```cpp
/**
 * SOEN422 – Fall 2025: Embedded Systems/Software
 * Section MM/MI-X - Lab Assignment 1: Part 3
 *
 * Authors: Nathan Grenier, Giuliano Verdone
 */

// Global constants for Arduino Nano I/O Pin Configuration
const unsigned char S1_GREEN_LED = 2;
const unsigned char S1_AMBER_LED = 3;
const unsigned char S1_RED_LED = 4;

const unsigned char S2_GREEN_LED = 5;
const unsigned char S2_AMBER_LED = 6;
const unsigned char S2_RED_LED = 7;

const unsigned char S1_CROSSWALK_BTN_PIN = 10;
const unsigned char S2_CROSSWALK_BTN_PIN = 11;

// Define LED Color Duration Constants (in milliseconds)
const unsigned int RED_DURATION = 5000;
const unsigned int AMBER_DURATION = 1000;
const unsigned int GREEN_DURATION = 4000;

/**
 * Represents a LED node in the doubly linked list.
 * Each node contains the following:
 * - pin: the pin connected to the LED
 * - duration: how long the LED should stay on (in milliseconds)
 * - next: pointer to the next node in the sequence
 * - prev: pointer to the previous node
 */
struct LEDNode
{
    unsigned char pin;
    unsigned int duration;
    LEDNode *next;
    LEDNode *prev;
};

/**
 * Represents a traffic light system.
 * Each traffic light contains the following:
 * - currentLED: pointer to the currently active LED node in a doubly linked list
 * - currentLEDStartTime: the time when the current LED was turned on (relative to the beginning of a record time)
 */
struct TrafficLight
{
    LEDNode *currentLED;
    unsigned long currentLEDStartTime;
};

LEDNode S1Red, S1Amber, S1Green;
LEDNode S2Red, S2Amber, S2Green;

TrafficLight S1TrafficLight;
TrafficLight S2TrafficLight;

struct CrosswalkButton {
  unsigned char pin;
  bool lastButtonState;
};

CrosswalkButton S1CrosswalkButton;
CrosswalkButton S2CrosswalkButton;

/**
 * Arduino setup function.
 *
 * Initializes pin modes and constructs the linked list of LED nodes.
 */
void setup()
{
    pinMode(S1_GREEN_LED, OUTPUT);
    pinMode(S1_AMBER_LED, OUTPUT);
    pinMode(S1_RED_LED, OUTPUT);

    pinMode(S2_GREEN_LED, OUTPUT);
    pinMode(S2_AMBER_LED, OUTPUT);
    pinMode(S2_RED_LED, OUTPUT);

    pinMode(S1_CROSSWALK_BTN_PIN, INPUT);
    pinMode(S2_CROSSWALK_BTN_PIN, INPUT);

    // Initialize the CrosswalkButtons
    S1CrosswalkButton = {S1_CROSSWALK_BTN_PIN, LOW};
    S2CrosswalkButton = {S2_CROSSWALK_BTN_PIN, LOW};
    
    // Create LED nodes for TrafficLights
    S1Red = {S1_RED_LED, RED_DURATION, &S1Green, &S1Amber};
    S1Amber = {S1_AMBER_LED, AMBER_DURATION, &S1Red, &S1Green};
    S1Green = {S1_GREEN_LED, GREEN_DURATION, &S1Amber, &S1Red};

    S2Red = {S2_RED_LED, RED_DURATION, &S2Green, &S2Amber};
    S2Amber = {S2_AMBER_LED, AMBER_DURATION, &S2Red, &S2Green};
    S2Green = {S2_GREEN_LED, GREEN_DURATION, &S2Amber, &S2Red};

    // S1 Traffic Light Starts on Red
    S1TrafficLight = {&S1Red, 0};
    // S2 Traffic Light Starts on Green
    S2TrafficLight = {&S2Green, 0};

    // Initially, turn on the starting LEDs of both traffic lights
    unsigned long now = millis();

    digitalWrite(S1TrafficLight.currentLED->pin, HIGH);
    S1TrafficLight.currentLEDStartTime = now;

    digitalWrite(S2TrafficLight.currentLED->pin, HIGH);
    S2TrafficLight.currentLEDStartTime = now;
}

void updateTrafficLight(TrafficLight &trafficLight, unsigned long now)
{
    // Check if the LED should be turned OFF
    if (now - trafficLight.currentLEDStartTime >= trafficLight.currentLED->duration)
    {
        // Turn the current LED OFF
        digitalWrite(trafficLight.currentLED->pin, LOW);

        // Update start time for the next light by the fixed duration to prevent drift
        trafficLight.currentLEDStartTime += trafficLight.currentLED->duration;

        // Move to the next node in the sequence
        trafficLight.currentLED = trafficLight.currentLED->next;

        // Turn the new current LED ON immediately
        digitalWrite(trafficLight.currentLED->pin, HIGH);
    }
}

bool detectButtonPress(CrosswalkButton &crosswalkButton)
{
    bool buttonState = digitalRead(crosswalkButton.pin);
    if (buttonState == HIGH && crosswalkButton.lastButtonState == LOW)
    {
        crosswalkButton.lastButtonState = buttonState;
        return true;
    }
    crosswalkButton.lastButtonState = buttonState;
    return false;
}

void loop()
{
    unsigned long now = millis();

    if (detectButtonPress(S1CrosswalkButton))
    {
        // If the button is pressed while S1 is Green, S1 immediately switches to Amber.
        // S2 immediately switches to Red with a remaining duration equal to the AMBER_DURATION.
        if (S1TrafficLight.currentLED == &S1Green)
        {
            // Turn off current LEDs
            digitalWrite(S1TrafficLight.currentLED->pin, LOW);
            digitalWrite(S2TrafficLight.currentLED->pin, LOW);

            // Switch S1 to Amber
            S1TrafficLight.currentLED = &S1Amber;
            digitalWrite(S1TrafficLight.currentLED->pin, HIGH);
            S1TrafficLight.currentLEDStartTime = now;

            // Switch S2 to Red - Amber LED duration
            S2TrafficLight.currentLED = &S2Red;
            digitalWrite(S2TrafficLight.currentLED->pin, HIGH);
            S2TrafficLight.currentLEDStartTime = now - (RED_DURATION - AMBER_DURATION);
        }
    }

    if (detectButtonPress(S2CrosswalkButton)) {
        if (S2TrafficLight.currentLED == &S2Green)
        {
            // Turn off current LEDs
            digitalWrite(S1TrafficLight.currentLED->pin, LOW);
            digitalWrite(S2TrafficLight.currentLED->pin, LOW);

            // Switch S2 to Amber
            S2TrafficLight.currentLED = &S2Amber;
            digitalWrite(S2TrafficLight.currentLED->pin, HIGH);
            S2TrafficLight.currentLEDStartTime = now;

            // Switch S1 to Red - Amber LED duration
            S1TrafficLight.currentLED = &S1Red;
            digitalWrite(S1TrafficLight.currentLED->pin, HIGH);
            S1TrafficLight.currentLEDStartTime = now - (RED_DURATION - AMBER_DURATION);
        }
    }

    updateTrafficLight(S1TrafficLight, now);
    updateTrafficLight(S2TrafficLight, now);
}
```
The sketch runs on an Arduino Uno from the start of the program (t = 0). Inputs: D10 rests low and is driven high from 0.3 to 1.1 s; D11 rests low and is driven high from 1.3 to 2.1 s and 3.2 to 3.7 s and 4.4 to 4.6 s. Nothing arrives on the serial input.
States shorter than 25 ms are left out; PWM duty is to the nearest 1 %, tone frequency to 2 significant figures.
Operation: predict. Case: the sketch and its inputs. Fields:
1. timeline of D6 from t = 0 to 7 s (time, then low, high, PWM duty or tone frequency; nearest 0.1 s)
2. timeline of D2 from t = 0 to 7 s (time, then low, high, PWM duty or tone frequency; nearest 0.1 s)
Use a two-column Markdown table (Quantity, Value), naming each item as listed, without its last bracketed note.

| Quantity | Value |
|---|---|
| timeline of D6 from t = 0 to 7 s | 0 s low; 1.3 s high; 2.3 s low |
| timeline of D2 from t = 0 to 7 s | 0 s low; 2.3 s high; 6.3 s low |
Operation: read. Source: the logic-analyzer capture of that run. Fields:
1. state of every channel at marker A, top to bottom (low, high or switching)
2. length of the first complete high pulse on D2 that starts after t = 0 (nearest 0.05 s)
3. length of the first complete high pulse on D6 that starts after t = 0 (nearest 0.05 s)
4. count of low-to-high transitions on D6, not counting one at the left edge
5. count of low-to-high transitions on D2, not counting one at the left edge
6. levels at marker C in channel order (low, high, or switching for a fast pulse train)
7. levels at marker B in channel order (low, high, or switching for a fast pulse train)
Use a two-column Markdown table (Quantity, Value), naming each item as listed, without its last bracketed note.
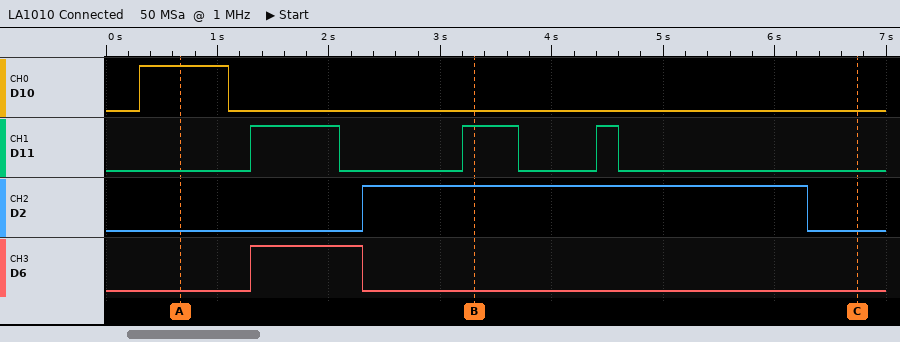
| Quantity | Value |
|---|---|
| state of every channel at marker A, top to bottom | D10 high, D11 low, D2 low, D6 low |
| length of the first complete high pulse on D2 that starts after t = 0 | 4.00 s |
| length of the first complete high pulse on D6 that starts after t = 0 | 1.00 s |
| count of low-to-high transitions on D6, not counting one at the left edge | 1 |
| count of low-to-high transitions on D2, not counting one at the left edge | 1 |
| levels at marker C in channel order | D10 low, D11 low, D2 low, D6 low |
| levels at marker B in channel order | D10 low, D11 high, D2 high, D6 low |
